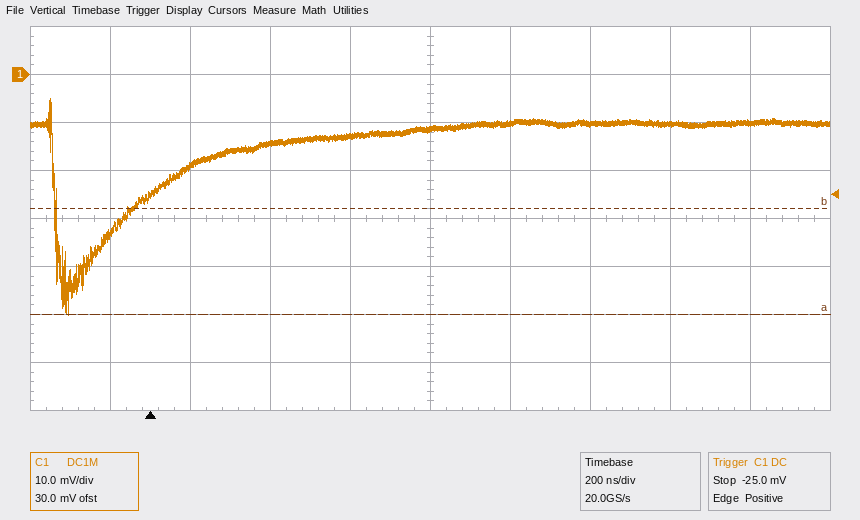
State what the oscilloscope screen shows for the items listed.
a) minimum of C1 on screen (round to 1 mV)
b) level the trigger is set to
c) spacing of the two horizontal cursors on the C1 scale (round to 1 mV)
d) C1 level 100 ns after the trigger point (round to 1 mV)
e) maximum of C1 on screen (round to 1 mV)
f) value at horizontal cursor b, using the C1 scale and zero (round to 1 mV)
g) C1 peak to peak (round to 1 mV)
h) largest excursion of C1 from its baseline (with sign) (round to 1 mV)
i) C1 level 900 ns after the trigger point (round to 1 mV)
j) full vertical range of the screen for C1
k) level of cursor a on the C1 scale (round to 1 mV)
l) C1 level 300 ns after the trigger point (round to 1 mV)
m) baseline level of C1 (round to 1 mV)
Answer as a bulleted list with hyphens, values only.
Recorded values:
- -50 mV
- -25.0 mV
- 22 mV
- -19 mV
- -5 mV
- -28 mV
- 45 mV
- -40 mV
- -10 mV
- 80 mV
- -50 mV
- -14 mV
- -10 mV
